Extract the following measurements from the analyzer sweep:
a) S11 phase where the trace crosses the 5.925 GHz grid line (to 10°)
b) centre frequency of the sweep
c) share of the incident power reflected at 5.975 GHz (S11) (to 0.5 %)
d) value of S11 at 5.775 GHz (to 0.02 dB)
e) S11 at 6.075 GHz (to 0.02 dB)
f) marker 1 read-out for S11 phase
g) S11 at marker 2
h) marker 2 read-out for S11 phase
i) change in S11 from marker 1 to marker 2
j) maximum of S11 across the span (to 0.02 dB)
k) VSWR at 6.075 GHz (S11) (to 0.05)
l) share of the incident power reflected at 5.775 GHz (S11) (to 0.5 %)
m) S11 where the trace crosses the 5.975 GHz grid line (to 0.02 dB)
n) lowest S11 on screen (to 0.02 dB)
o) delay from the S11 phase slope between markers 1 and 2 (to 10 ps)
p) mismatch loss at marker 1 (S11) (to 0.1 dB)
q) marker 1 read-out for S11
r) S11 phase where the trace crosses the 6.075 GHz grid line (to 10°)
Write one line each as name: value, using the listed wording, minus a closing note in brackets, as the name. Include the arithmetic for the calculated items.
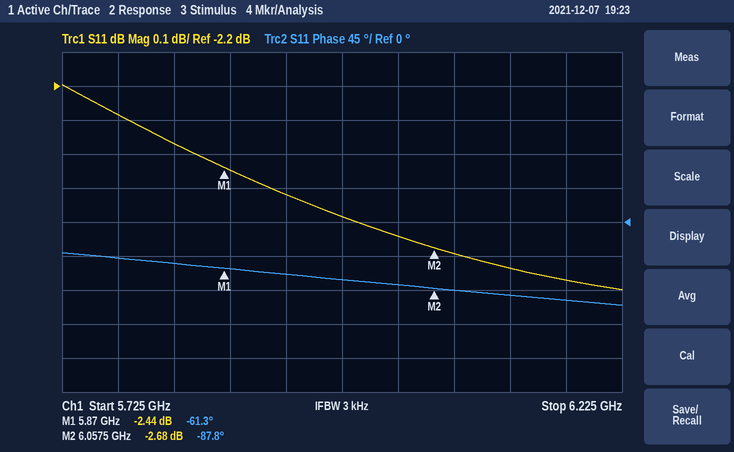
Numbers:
S11 phase where the trace crosses the 5.925 GHz grid line: -70°
centre frequency of the sweep: 5.975 GHz
share of the incident power reflected at 5.975 GHz (S11): 10^(-2.58/10) ≈ 55.2 %, so 55.0 % to the nearest 0.5 %
value of S11 at 5.775 GHz: -2.28 dB
S11 at 6.075 GHz: -2.70 dB
marker 1 read-out for S11 phase: -61.3°
S11 at marker 2: -2.68 dB
marker 2 read-out for S11 phase: -87.8°
change in S11 from marker 1 to marker 2: -2.68 − (-2.44) = -0.24 dB
maximum of S11 across the span: -2.20 dB
VSWR at 6.075 GHz (S11): |Γ| = 10^(-2.7/20) = 0.7328; VSWR = (1 + 0.7328)/(1 − 0.7328) ≈ 6.49, so 6.50 to the nearest 0.05
share of the incident power reflected at 5.775 GHz (S11): 10^(-2.28/10) ≈ 59.2 %, so 59.0 % to the nearest 0.5 %
S11 where the trace crosses the 5.975 GHz grid line: -2.58 dB
lowest S11 on screen: -2.80 dB
delay from the S11 phase slope between markers 1 and 2: −(-87.8° − (-61.3°))/(360° × 187.5 MHz) ≈ 393 ps, so 390 ps to the nearest 10 ps
mismatch loss at marker 1 (S11): −10 log10(1 − 10^(-2.44/10)) ≈ 3.7 dB
marker 1 read-out for S11: -2.44 dB
S11 phase where the trace crosses the 6.075 GHz grid line: -90°
